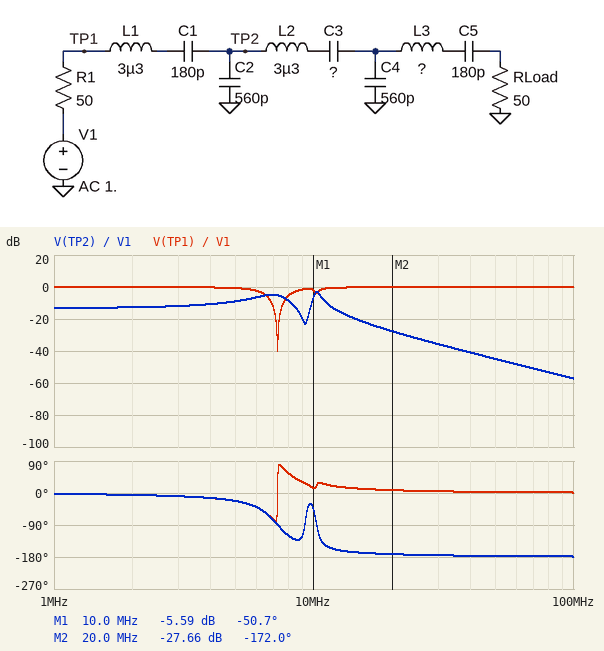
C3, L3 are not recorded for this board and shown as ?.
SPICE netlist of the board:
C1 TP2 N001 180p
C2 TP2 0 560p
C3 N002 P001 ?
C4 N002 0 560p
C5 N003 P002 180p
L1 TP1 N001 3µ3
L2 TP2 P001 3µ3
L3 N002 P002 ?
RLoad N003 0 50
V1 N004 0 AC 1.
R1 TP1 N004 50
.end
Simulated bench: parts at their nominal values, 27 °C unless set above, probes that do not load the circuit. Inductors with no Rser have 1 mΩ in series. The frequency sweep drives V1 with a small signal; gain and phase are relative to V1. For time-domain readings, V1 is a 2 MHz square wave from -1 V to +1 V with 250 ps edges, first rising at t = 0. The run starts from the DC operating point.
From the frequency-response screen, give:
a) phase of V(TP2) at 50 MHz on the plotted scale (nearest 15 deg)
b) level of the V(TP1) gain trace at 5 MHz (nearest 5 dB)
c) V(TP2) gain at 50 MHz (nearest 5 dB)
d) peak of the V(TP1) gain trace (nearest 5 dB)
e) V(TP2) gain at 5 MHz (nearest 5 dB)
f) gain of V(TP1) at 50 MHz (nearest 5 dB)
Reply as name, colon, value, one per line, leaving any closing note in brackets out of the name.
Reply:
phase of V(TP2) at 50 MHz on the plotted scale: -180 deg
level of the V(TP1) gain trace at 5 MHz: 0 dB
V(TP2) gain at 50 MHz: -45 dB
peak of the V(TP1) gain trace: 0 dB
V(TP2) gain at 5 MHz: -10 dB
gain of V(TP1) at 50 MHz: 0 dB
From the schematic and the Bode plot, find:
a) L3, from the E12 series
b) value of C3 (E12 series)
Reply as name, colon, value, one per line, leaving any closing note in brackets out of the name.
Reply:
L3, from the E12 series: 1.2 µH
value of C3: 100 pF
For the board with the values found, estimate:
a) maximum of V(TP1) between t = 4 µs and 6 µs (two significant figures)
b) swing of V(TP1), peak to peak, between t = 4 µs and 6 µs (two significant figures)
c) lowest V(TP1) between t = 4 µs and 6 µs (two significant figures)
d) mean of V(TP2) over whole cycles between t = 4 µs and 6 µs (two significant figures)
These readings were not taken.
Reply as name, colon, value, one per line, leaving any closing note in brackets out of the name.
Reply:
maximum of V(TP1) between t = 4 µs and 6 µs: 1.2 V
swing of V(TP1), peak to peak, between t = 4 µs and 6 µs: 2.5 V
lowest V(TP1) between t = 4 µs and 6 µs: -1.2 V
mean of V(TP2) over whole cycles between t = 4 µs and 6 µs: 220 mV
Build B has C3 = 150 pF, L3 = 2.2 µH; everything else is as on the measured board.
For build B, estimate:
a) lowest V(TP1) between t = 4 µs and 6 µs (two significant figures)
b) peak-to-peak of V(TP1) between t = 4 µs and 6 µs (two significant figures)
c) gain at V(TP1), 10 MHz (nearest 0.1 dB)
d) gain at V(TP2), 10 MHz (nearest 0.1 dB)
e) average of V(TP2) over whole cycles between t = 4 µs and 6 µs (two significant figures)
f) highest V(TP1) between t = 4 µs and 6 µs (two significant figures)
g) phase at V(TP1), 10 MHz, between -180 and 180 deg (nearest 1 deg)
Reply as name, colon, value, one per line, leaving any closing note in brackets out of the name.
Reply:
lowest V(TP1) between t = 4 µs and 6 µs: -1.3 V
peak-to-peak of V(TP1) between t = 4 µs and 6 µs: 2.6 V
gain at V(TP1), 10 MHz: -2.1 dB
gain at V(TP2), 10 MHz: -5.7 dB
average of V(TP2) over whole cycles between t = 4 µs and 6 µs: 210 mV
highest V(TP1) between t = 4 µs and 6 µs: 1.3 V
phase at V(TP1), 10 MHz, between -180 and 180 deg: 33 deg
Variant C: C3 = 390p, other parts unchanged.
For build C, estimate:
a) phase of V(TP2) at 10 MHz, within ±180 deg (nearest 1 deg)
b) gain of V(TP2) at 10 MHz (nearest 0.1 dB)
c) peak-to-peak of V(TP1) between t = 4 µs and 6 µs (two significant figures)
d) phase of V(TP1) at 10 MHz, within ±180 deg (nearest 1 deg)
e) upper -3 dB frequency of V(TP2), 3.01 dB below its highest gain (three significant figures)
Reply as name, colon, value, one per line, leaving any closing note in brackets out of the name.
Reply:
phase of V(TP2) at 10 MHz, within ±180 deg: -148 deg
gain of V(TP2) at 10 MHz: -8.9 dB
peak-to-peak of V(TP1) between t = 4 µs and 6 µs: 2.5 V
phase of V(TP1) at 10 MHz, within ±180 deg: 31 deg
upper -3 dB frequency of V(TP2), 3.01 dB below its highest gain: 8.60 MHz
